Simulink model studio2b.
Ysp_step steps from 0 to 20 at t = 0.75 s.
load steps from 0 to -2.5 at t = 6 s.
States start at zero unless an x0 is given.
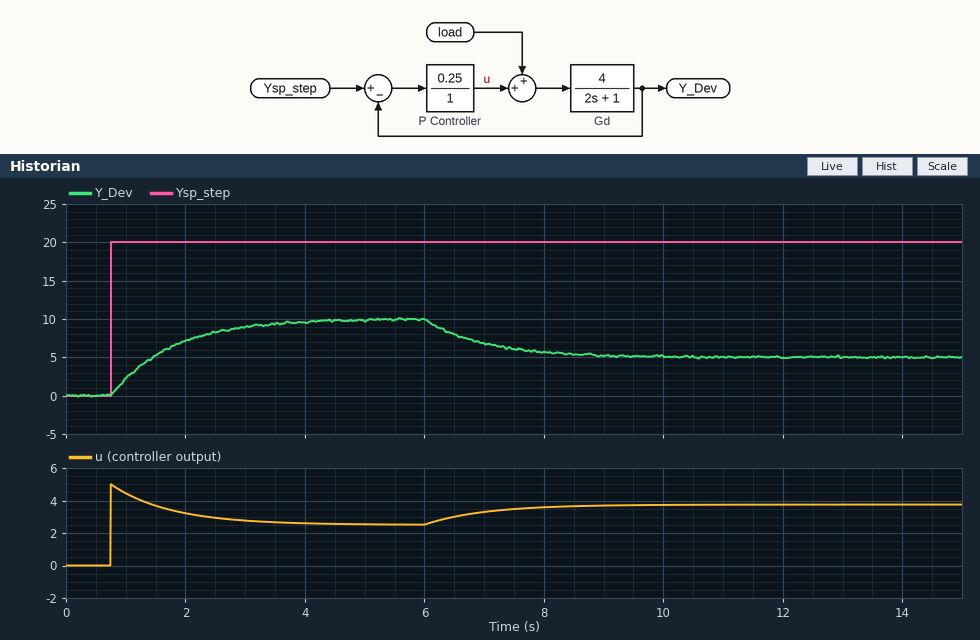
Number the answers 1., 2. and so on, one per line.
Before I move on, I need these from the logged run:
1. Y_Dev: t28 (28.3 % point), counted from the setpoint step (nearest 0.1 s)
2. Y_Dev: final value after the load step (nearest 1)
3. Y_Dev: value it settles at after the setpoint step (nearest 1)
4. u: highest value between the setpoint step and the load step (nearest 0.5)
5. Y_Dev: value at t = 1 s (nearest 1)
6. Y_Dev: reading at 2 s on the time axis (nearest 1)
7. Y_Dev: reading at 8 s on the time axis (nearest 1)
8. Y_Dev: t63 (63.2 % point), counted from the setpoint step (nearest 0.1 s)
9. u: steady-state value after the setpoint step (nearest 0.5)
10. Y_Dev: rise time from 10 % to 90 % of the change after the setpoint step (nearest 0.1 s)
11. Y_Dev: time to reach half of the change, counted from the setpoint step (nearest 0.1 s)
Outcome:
1. 0.3 s
2. 5
3. 10
4. 5.0
5. 2
6. 7
7. 6
8. 1.0 s
9. 2.5
10. 2.2 s
11. 0.7 s
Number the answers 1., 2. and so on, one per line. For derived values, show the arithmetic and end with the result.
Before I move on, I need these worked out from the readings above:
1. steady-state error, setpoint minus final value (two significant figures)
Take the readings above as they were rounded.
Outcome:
1. 20 - 10 = 10
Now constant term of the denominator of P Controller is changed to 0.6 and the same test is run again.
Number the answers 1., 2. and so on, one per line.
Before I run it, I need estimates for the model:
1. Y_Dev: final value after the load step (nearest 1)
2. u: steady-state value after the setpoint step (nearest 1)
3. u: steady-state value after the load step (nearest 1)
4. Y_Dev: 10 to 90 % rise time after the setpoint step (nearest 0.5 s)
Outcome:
1. 9
2. 3
3. 5
4. 1.5 s
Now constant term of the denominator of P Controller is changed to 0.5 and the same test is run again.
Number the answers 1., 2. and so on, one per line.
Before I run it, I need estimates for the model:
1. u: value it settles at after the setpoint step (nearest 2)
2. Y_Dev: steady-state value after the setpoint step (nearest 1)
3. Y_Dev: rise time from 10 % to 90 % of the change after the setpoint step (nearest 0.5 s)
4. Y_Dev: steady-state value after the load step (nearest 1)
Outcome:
1. 4
2. 13
3. 1.5 s
4. 10
